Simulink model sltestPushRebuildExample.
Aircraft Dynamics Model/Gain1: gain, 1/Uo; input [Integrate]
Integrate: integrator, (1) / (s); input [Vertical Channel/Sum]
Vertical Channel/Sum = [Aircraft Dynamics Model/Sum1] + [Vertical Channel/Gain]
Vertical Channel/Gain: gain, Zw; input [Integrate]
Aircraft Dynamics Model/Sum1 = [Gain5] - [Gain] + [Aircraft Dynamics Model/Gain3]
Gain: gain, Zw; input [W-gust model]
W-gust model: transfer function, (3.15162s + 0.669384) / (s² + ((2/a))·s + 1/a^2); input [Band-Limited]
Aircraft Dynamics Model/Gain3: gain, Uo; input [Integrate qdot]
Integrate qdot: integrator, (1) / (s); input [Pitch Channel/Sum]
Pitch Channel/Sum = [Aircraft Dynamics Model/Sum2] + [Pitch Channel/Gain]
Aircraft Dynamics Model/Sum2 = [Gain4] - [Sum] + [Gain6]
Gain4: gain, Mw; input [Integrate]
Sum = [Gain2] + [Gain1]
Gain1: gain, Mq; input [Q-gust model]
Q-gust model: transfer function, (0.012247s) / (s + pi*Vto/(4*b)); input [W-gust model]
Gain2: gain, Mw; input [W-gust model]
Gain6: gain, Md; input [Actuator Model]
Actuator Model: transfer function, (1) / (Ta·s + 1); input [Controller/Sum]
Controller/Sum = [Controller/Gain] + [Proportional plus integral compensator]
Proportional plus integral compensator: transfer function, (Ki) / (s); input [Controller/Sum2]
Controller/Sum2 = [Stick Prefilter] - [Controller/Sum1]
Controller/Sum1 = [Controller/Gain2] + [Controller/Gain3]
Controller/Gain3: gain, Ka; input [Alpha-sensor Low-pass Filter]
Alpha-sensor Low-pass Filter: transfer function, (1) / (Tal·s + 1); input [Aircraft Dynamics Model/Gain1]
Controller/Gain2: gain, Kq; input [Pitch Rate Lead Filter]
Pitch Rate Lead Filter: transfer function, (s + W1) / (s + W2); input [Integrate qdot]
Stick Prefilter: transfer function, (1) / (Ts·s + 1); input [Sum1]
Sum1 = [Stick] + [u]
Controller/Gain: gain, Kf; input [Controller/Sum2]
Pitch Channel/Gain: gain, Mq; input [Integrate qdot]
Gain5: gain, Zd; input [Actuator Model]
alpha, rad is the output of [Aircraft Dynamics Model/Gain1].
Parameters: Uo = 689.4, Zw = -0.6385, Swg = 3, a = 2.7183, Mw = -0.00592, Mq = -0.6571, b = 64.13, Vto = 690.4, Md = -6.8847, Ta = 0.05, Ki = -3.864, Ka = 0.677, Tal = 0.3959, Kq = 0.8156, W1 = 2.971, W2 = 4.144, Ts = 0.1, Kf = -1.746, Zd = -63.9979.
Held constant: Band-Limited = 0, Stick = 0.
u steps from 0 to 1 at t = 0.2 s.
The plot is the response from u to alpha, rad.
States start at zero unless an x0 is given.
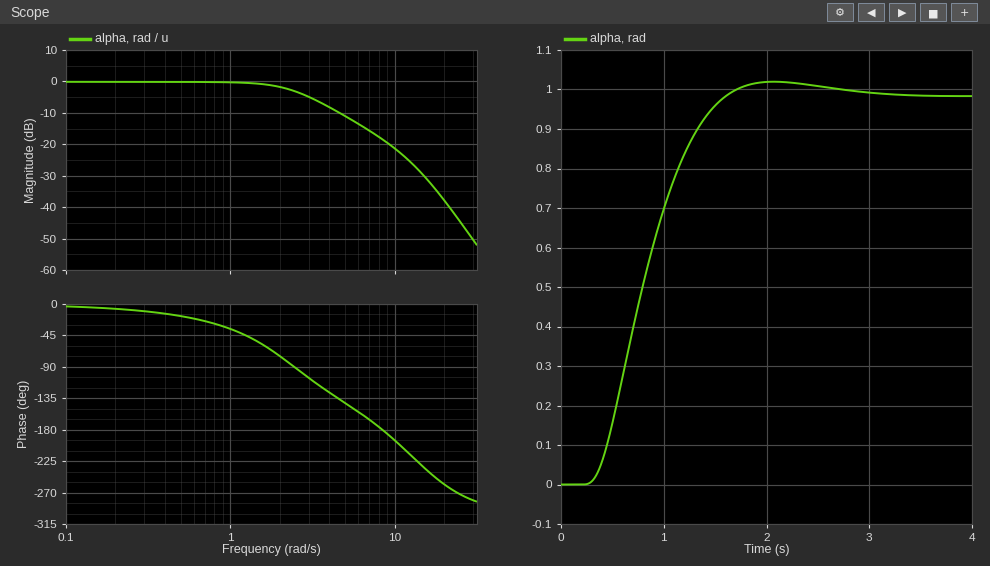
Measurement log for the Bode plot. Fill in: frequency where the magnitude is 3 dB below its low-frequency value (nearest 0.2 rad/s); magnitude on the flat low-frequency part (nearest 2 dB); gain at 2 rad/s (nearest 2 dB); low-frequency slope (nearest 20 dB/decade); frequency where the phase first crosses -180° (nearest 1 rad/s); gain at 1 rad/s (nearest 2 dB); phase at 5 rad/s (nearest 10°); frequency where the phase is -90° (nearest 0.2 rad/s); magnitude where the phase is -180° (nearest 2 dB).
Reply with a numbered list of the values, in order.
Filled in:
1. 2.4 rad/s
2. 0 dB
3. -2 dB
4. 0 dB/decade
5. 8 rad/s
6. 0 dB
7. -140°
8. 2.4 rad/s
9. -18 dB
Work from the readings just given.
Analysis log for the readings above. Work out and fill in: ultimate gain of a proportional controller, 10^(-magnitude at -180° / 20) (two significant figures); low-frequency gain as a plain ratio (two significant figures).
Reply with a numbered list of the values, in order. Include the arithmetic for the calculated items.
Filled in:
1. 10^(18 / 20) = 7.9
2. 10^(0 / 20) = 1.0
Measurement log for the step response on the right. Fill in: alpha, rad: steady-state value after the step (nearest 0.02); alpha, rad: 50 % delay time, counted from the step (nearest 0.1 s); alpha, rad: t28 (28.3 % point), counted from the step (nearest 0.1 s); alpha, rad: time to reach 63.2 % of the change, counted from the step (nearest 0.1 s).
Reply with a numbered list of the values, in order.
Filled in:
1. 0.98
2. 0.6 s
3. 0.4 s
4. 0.7 s
